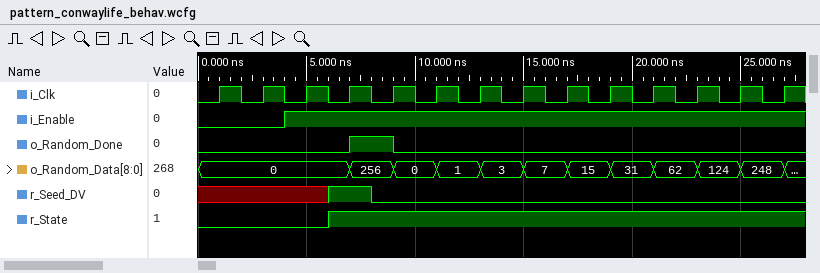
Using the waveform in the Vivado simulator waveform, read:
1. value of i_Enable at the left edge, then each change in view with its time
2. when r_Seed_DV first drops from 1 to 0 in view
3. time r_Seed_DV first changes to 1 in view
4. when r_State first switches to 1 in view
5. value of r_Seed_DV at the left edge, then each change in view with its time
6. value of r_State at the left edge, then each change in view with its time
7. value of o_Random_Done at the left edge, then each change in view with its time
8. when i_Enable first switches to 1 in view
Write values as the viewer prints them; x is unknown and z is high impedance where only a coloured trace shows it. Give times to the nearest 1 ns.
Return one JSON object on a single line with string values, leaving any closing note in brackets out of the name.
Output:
{"value of i_Enable at the left edge, then each change in view with its time": "0, 1 at 4 ns", "when r_Seed_DV first drops from 1 to 0 in view": "8 ns", "time r_Seed_DV first changes to 1 in view": "6 ns", "when r_State first switches to 1 in view": "6 ns", "value of r_Seed_DV at the left edge, then each change in view with its time": "x, 1 at 6 ns, 0 at 8 ns", "value of r_State at the left edge, then each change in view with its time": "0, 1 at 6 ns", "value of o_Random_Done at the left edge, then each change in view with its time": "0, 1 at 7 ns, 0 at 9 ns", "when i_Enable first switches to 1 in view": "4 ns"}
